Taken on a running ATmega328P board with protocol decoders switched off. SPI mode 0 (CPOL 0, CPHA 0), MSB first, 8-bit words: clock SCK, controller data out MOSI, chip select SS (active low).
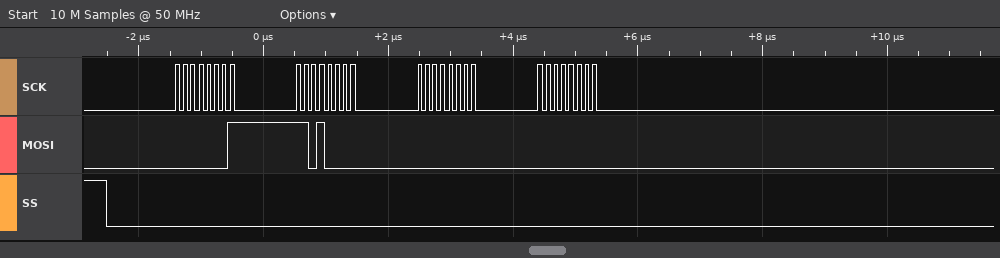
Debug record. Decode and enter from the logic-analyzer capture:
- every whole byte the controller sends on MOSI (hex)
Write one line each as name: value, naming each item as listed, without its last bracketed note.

every whole byte the controller sends on MOSI: 01 D0 00 00
